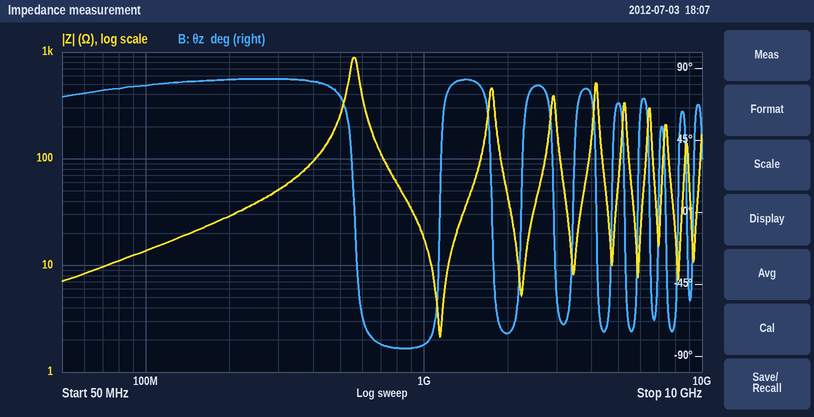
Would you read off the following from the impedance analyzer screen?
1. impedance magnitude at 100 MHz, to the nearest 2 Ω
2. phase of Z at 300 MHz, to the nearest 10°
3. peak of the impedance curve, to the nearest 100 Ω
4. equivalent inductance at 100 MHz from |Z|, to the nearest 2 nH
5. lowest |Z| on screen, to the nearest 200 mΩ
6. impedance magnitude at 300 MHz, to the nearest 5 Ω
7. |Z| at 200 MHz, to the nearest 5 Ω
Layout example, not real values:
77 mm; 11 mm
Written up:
14 Ω; 80°; 900 Ω; 22 nH; 2.2 Ω; 50 Ω; 30 Ω
